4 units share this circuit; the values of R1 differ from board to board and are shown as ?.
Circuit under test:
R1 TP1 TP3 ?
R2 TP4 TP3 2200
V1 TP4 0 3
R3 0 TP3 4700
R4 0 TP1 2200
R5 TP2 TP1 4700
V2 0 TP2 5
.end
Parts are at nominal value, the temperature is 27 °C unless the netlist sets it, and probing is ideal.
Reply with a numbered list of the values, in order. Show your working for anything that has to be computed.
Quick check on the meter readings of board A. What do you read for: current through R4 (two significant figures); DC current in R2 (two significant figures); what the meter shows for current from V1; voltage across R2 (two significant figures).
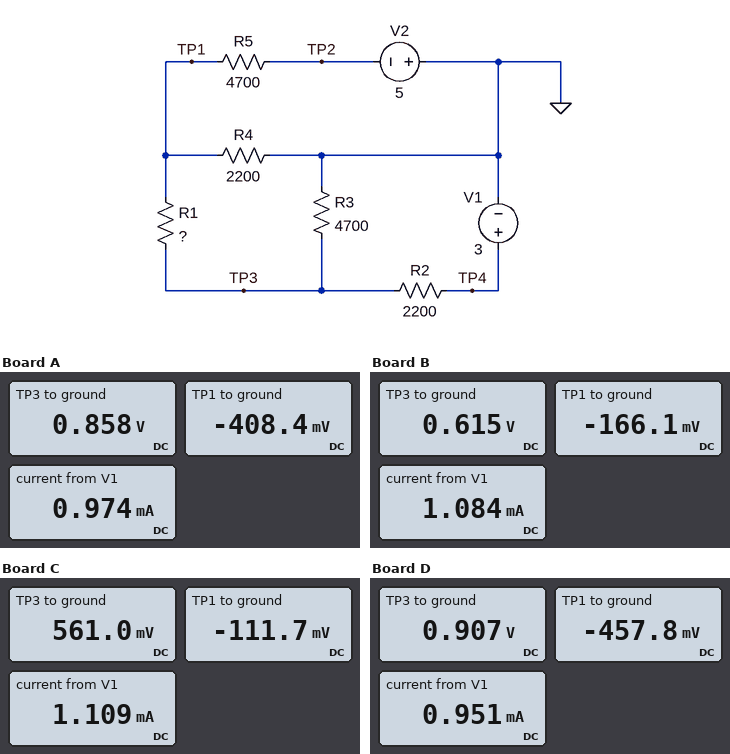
1. (0 V - (-408.4 mV)) / 2.2 kΩ = 190 µA
2. (3 V - 858 mV) / 2.2 kΩ = 970 µA
3. 0.974 mA
4. 3 V - 858 mV = 2.1 V
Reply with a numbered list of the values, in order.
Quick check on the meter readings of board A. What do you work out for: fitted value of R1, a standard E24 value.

1. 1.6 kΩ
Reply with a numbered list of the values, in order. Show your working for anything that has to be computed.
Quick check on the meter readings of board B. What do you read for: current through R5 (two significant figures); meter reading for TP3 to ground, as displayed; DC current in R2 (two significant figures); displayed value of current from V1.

1. (-166.1 mV - (-5 V)) / 4.7 kΩ = 1.0 mA
2. 0.615 V
3. (3 V - 615 mV) / 2.2 kΩ = 1.1 mA
4. 1.084 mA
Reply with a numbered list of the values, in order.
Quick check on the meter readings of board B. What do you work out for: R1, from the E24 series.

1. 820 Ω
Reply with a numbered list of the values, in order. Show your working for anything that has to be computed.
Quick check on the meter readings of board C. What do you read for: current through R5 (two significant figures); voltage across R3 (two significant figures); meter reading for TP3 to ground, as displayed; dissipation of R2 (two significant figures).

1. (-111.7 mV - (-5 V)) / 4.7 kΩ = 1.0 mA
2. 561 mV = 560 mV
3. 561.0 mV
4. (3 V - 561 mV)^2 / 2.2 kΩ = 2.7 mW
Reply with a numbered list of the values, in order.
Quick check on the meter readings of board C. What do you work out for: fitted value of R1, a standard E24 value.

1. 680 Ω
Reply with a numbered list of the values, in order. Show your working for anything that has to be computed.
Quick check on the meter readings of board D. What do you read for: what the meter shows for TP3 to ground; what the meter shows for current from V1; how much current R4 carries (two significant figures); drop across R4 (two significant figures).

1. 0.907 V
2. 0.951 mA
3. (0 V - (-457.8 mV)) / 2.2 kΩ = 210 µA
4. 0 V - (-457.8 mV) = 460 mV
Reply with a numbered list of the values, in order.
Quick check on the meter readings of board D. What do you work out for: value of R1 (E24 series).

1. 1.8 kΩ
